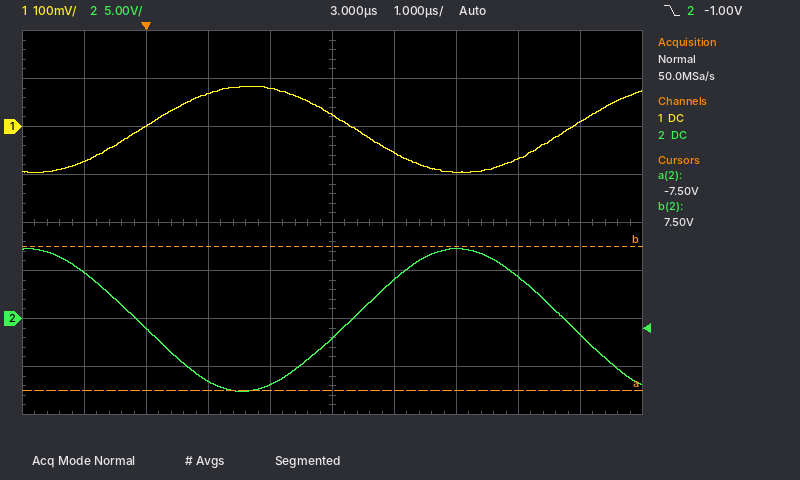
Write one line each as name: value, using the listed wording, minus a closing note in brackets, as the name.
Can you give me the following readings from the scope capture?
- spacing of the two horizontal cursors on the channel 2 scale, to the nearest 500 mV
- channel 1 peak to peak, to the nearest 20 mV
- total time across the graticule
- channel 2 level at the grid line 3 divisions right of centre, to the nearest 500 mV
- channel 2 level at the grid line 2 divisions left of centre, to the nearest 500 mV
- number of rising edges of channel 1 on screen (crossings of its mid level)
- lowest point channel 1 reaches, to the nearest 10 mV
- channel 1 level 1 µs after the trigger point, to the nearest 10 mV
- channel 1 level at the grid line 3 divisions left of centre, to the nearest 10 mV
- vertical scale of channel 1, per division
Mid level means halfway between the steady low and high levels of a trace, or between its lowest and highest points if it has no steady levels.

spacing of the two horizontal cursors on the channel 2 scale, to the nearest 500 mV: 15.0 V
channel 1 peak to peak, to the nearest 20 mV: 180 mV
total time across the graticule: 10 µs
channel 2 level at the grid line 3 divisions right of centre, to the nearest 500 mV: 4.5 V
channel 2 level at the grid line 2 divisions left of centre, to the nearest 500 mV: -6.5 V
number of rising edges of channel 1 on screen: 2
lowest point channel 1 reaches, to the nearest 10 mV: -100 mV
channel 1 level 1 µs after the trigger point, to the nearest 10 mV: 70 mV
channel 1 level at the grid line 3 divisions left of centre, to the nearest 10 mV: 0 mV
vertical scale of channel 1, per division: 100 mV
